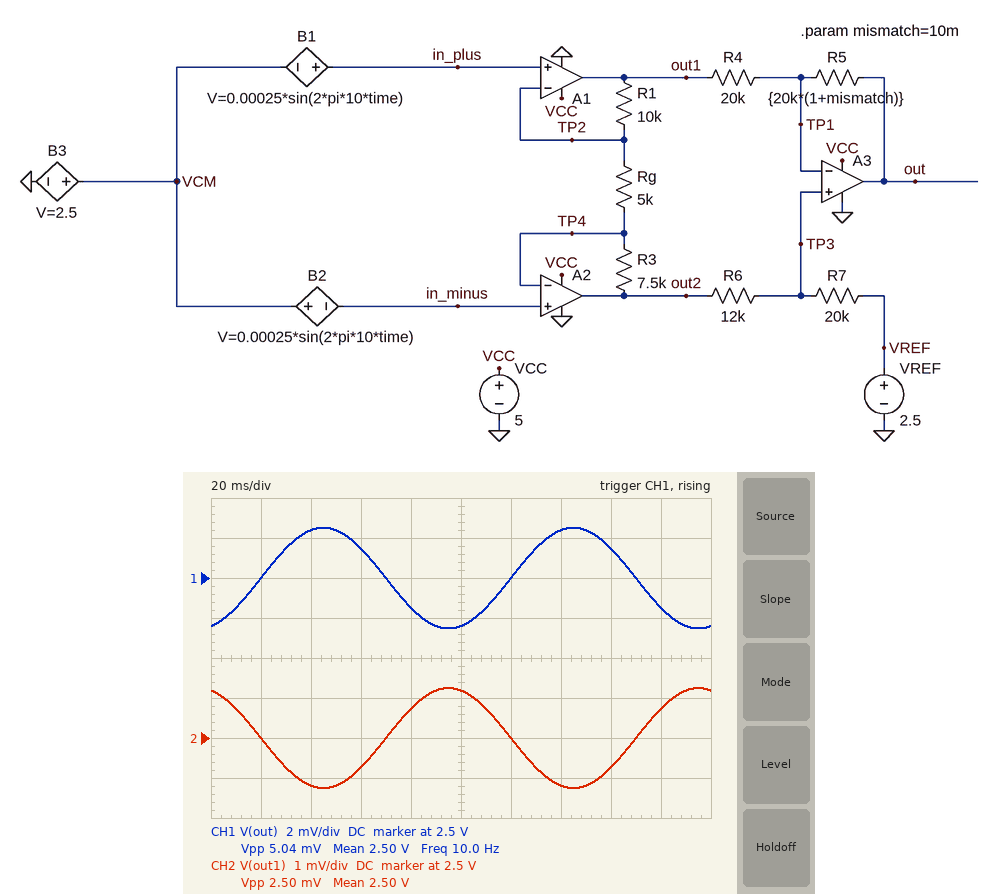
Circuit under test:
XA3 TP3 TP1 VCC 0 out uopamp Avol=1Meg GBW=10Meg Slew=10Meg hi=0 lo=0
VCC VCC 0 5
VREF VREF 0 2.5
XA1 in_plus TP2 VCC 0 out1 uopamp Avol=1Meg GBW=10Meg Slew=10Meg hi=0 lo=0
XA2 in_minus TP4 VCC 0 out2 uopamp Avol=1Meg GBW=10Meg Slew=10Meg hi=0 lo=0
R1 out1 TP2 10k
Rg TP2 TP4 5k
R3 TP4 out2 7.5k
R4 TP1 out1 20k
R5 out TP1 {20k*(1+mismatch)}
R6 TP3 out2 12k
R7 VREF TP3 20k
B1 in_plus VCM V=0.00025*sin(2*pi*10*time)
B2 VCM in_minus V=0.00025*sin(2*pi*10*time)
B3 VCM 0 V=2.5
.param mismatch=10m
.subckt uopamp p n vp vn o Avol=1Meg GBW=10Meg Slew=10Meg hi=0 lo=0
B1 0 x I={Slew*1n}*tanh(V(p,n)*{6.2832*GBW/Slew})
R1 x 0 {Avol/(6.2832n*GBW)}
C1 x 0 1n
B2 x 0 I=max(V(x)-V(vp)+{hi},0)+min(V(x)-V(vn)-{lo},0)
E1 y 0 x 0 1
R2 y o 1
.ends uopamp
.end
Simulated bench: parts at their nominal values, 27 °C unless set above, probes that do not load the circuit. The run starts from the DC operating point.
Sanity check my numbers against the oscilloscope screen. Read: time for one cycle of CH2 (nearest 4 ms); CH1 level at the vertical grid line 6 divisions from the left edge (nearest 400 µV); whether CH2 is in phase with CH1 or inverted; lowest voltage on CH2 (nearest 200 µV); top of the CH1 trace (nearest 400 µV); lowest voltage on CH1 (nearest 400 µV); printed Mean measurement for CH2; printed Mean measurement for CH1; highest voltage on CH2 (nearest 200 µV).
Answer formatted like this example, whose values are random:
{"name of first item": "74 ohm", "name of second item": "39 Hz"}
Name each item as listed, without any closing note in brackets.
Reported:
{"time for one cycle of CH2": "100 ms", "CH1 level at the vertical grid line 6 divisions from the left edge": "2.5000 V", "whether CH2 is in phase with CH1 or inverted": "inverted", "lowest voltage on CH2": "2.4988 V", "top of the CH1 trace": "2.5024 V", "lowest voltage on CH1": "2.4976 V", "printed Mean measurement for CH2": "2.50 V", "printed Mean measurement for CH1": "2.50 V", "highest voltage on CH2": "2.5012 V"}
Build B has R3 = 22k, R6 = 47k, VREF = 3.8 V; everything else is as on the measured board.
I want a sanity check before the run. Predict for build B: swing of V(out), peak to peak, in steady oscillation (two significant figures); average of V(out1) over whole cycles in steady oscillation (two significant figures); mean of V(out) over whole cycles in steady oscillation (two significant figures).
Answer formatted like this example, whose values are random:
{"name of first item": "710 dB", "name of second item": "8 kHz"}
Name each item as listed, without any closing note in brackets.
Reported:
{"swing of V(out), peak to peak, in steady oscillation": "5.5 mV", "average of V(out1) over whole cycles in steady oscillation": "2.5 V", "mean of V(out) over whole cycles in steady oscillation": "4.3 V"}
